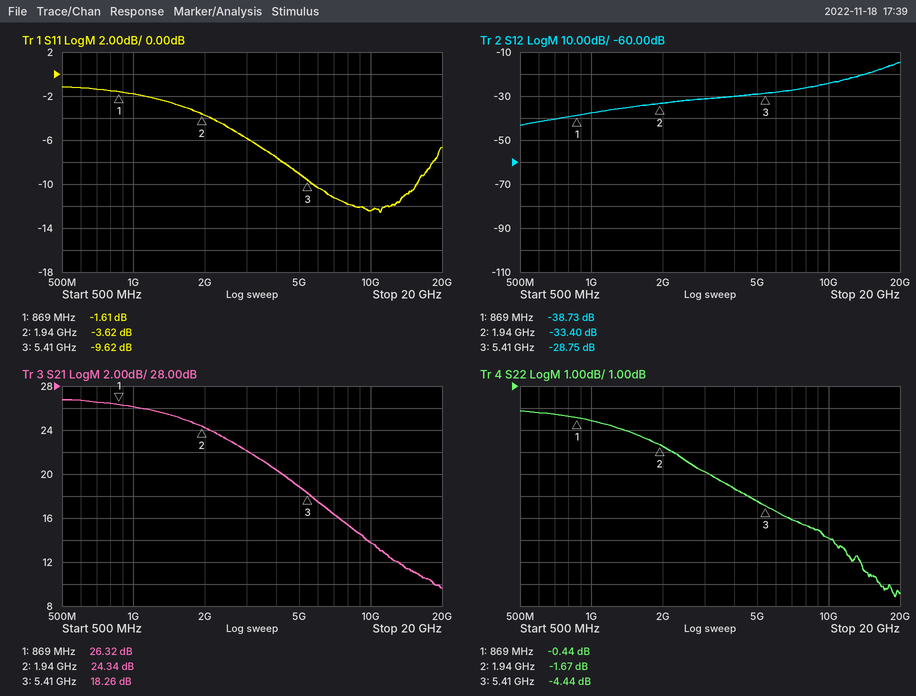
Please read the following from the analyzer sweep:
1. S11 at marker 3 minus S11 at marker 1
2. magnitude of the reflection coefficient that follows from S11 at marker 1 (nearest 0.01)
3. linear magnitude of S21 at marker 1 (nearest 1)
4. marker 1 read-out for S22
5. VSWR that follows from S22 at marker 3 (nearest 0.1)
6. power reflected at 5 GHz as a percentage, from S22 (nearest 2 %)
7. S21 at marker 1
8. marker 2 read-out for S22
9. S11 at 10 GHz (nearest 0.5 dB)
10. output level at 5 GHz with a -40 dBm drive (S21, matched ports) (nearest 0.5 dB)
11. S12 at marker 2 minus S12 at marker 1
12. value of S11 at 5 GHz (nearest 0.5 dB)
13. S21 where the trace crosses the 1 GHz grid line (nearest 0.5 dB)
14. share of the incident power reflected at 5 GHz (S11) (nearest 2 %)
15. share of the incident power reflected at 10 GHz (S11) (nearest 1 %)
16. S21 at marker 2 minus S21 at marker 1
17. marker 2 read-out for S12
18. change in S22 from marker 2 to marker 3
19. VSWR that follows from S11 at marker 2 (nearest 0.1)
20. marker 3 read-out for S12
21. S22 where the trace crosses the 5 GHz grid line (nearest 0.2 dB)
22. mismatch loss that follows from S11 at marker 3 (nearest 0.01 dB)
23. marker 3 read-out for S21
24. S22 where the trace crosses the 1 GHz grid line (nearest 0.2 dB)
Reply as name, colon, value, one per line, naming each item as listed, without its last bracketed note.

S11 at marker 3 minus S11 at marker 1: -8.01 dB
magnitude of the reflection coefficient that follows from S11 at marker 1: 0.83
linear magnitude of S21 at marker 1: 21
marker 1 read-out for S22: -0.44 dB
VSWR that follows from S22 at marker 3: 4.0
power reflected at 5 GHz as a percentage, from S22: 38 %
S21 at marker 1: 26.32 dB
marker 2 read-out for S22: -1.67 dB
S11 at 10 GHz: -12.5 dB
output level at 5 GHz with a -40 dBm drive (S21, matched ports): -21.0 dBm
S12 at marker 2 minus S12 at marker 1: 5.33 dB
value of S11 at 5 GHz: -9.0 dB
S21 where the trace crosses the 1 GHz grid line: 26.0 dB
share of the incident power reflected at 5 GHz (S11): 12 %
share of the incident power reflected at 10 GHz (S11): 6 %
S21 at marker 2 minus S21 at marker 1: -1.98 dB
marker 2 read-out for S12: -33.40 dB
change in S22 from marker 2 to marker 3: -2.77 dB
VSWR that follows from S11 at marker 2: 4.9
marker 3 read-out for S12: -28.75 dB
S22 where the trace crosses the 5 GHz grid line: -4.2 dB
mismatch loss that follows from S11 at marker 3: 0.50 dB
marker 3 read-out for S21: 18.26 dB
S22 where the trace crosses the 1 GHz grid line: -0.6 dB
